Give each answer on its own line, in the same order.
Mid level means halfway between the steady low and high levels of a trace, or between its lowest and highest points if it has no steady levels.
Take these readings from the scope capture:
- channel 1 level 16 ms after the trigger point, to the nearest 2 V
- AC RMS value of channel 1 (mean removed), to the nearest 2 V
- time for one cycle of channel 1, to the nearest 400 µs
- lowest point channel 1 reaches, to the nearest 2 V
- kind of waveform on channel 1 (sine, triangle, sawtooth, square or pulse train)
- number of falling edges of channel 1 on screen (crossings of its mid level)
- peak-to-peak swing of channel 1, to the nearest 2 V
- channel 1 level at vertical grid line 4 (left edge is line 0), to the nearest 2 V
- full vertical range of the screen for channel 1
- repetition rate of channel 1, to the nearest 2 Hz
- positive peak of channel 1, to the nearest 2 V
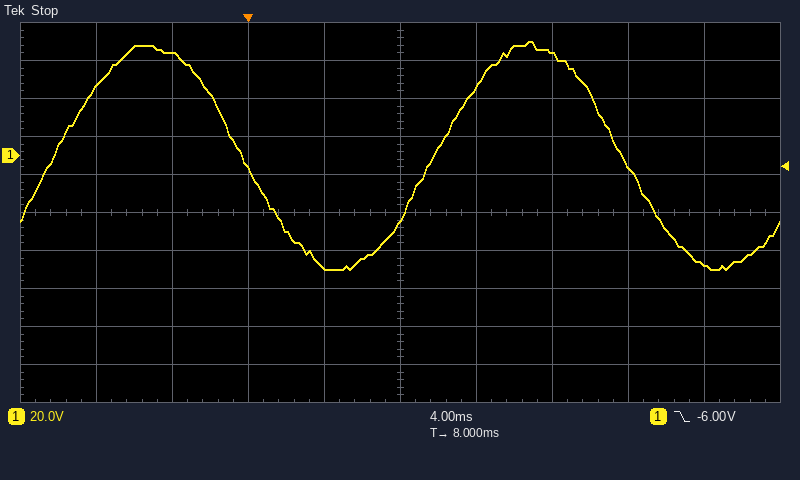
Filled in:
54 V
42 V
20.0 ms
-60 V
sine
2
120 V
-58 V
200 V
50 Hz
60 V
